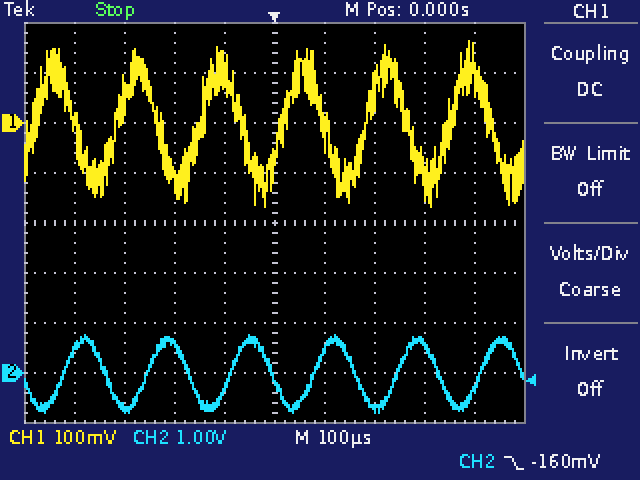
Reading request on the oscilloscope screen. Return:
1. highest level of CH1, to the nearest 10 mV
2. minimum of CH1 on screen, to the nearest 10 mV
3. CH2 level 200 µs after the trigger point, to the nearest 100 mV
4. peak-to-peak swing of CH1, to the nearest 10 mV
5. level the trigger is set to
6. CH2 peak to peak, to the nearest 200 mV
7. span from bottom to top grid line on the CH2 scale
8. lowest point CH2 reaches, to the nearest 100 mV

160 mV
-170 mV
-700 mV
330 mV
-160 mV
1.6 V
8 V
-800 mV
